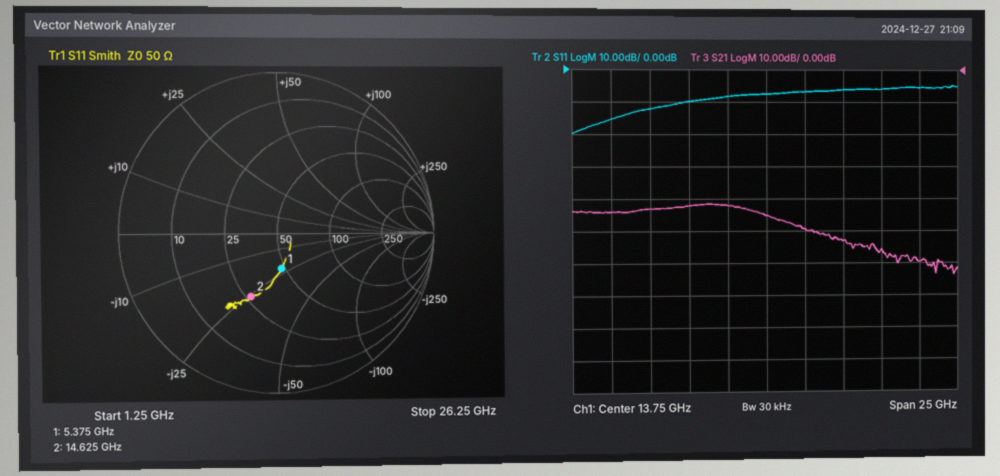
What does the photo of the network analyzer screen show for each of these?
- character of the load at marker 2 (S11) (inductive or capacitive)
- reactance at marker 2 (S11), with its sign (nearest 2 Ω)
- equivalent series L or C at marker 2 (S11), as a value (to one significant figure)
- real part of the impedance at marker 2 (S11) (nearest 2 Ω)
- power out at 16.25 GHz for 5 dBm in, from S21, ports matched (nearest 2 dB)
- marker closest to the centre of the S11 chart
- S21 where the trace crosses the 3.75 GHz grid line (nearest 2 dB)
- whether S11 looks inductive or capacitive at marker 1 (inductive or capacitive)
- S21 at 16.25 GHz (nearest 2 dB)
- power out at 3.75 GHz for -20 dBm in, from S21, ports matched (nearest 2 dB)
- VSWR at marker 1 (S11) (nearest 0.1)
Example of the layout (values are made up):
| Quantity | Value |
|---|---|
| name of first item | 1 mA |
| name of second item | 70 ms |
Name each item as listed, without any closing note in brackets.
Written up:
| Quantity | Value |
|---|---|
| character of the load at marker 2 (S11) | capacitive |
| reactance at marker 2 (S11), with its sign | -26 Ω |
| equivalent series L or C at marker 2 (S11), as a value | 400 fF |
| real part of the impedance at marker 2 (S11) | 26 Ω |
| power out at 16.25 GHz for 5 dBm in, from S21, ports matched | -44 dBm |
| marker closest to the centre of the S11 chart | marker 1 |
| S21 where the trace crosses the 3.75 GHz grid line | -44 dB |
| whether S11 looks inductive or capacitive at marker 1 | capacitive |
| S21 at 16.25 GHz | -50 dB |
| power out at 3.75 GHz for -20 dBm in, from S21, ports matched | -64 dBm |
| VSWR at marker 1 (S11) | 1.6 |
